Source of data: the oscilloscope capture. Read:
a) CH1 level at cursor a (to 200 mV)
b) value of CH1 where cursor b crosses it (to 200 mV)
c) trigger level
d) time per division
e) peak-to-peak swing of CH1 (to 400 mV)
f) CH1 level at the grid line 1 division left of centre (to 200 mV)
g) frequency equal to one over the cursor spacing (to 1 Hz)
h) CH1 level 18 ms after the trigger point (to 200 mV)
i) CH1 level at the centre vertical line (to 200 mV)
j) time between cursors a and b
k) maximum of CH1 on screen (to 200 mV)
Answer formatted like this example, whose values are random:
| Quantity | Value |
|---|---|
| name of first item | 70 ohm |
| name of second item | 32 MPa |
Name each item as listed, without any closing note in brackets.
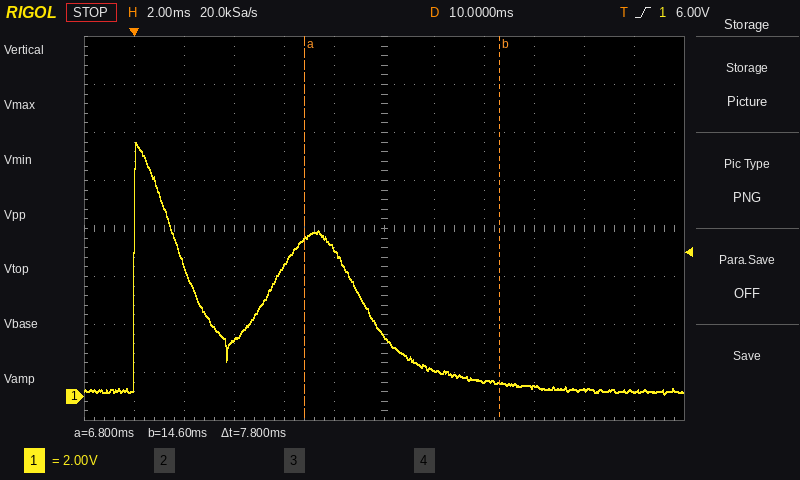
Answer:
| Quantity | Value |
|---|---|
| CH1 level at cursor a | 6.6 V |
| value of CH1 where cursor b crosses it | 600 mV |
| trigger level | 6.00 V |
| time per division | 2 ms |
| peak-to-peak swing of CH1 | 10.4 V |
| CH1 level at the grid line 1 division left of centre | 6.2 V |
| frequency equal to one over the cursor spacing | 128 Hz |
| CH1 level 18 ms after the trigger point | 200 mV |
| CH1 level at the centre vertical line | 2.6 V |
| time between cursors a and b | 7.8 ms |
| maximum of CH1 on screen | 10.6 V |
